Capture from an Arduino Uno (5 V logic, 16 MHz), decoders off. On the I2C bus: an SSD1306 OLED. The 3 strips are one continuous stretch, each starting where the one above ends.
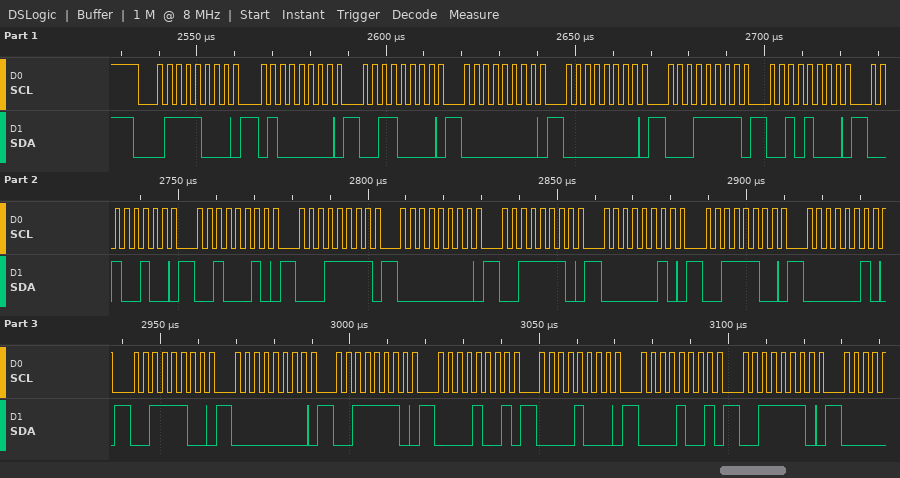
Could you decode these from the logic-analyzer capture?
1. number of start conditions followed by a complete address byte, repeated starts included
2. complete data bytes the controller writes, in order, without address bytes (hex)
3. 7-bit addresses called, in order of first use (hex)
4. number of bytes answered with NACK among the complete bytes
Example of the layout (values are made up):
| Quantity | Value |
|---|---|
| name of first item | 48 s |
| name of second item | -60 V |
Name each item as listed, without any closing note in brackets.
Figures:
| Quantity | Value |
|---|---|
| number of start conditions followed by a complete address byte, repeated starts included | 1 |
| complete data bytes the controller writes, in order, without address bytes | 40 30 00 00 1F 28 24 22 1F 00 3E 02 3C 02 3C 00 3E 09 08 09 3E |
| 7-bit addresses called, in order of first use | 0x3C |
| number of bytes answered with NACK among the complete bytes | 0 |
